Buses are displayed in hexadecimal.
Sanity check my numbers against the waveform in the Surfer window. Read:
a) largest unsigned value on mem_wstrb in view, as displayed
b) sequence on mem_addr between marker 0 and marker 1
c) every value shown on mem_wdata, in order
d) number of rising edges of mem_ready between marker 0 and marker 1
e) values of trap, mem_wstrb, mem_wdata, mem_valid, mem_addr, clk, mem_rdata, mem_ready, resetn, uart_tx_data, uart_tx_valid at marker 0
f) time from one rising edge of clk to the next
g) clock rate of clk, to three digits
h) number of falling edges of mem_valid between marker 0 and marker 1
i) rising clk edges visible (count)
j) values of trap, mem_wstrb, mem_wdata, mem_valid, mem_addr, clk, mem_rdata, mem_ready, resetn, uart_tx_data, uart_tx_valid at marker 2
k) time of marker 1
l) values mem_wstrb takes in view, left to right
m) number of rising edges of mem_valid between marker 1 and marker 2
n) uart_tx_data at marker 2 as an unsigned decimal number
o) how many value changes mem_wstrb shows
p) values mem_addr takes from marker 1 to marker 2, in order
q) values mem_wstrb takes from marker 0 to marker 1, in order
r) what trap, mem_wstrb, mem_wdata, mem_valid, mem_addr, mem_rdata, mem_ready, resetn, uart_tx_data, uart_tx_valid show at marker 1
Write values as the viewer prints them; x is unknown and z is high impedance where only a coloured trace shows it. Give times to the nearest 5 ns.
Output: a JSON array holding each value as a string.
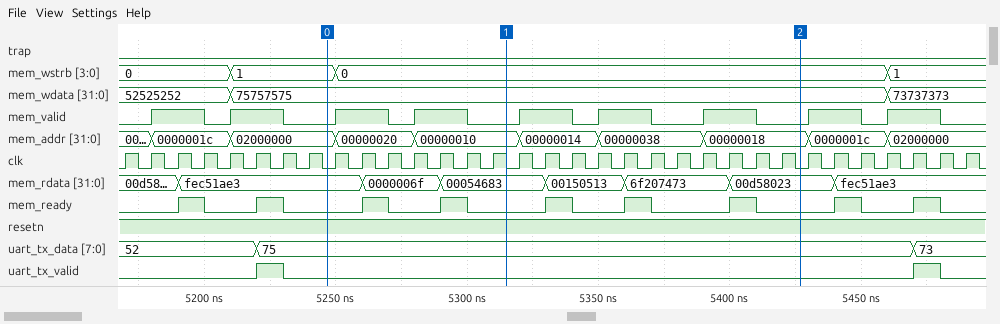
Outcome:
["1", "02000000, 00000020, 00000010", "52525252, 75757575, 73737373", "2", "trap=0, mem_wstrb=1, mem_wdata=75757575, mem_valid=0, mem_addr=02000000, clk=0, mem_rdata=fec51ae3, mem_ready=0, resetn=1, uart_tx_data=75, uart_tx_valid=0", "10 ns", "100 MHz", "2", "33", "trap=0, mem_wstrb=0, mem_wdata=75757575, mem_valid=0, mem_addr=00000018, clk=0, mem_rdata=00d58023, mem_ready=0, resetn=1, uart_tx_data=75, uart_tx_valid=0", "5315 ns", "0, 1, 0, 1", "3", "117", "3", "00000010, 00000014, 00000038, 00000018", "1, 0", "trap=0, mem_wstrb=0, mem_wdata=75757575, mem_valid=0, mem_addr=00000010, mem_rdata=00054683, mem_ready=0, resetn=1, uart_tx_data=75, uart_tx_valid=0"]
